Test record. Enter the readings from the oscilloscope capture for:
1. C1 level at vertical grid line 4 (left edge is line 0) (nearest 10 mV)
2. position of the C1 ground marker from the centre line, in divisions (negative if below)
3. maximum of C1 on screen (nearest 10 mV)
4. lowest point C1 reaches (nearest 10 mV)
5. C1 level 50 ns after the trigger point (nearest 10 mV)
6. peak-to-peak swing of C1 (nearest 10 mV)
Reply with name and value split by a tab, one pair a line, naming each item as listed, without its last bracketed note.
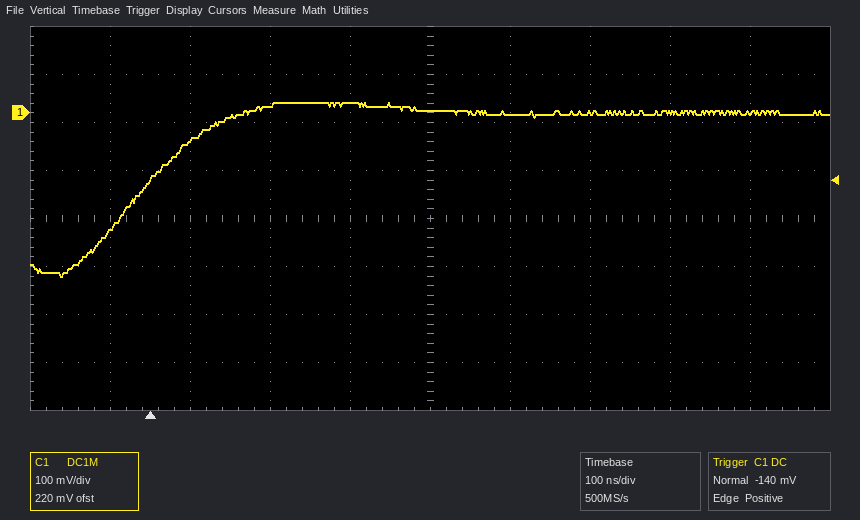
C1 level at vertical grid line 4 (left edge is line 0)	20 mV
position of the C1 ground marker from the centre line, in divisions	+2.2 div
maximum of C1 on screen	20 mV
lowest point C1 reaches	-340 mV
C1 level 50 ns after the trigger point	-60 mV
peak-to-peak swing of C1	360 mV
